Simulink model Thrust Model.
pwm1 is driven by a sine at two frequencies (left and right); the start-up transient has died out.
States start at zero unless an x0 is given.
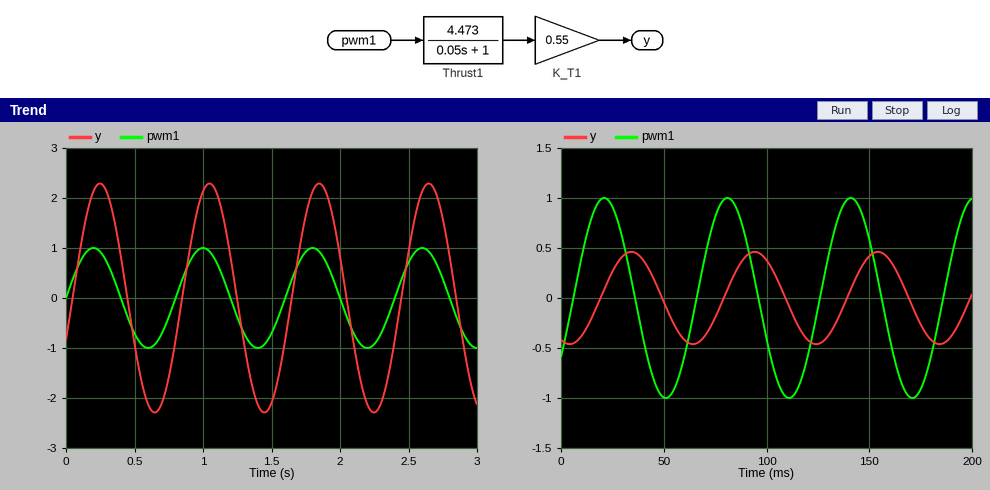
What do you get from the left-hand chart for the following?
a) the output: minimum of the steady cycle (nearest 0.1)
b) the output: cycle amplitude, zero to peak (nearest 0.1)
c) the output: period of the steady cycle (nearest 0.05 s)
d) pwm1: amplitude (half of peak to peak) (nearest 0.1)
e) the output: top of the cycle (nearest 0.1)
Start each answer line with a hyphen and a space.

- -2.3
- 2.3
- 0.80 s
- 1.0
- 2.3
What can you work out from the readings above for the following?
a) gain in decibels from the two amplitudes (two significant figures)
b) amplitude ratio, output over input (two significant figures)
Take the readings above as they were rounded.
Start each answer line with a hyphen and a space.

- 7.2 dB
- 2.3
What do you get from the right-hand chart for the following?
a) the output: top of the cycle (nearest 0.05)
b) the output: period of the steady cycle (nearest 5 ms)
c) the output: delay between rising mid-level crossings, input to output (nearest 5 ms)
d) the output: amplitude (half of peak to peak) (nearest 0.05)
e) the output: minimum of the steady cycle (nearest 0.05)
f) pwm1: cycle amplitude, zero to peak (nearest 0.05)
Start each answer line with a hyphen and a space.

- 0.45
- 60 ms
- 15 ms
- 0.45
- -0.45
- 1.00
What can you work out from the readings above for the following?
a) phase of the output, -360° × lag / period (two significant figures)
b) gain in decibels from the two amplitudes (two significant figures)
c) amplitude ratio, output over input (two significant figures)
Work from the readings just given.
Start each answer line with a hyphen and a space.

- -90°
- -6.9 dB
- 0.45
